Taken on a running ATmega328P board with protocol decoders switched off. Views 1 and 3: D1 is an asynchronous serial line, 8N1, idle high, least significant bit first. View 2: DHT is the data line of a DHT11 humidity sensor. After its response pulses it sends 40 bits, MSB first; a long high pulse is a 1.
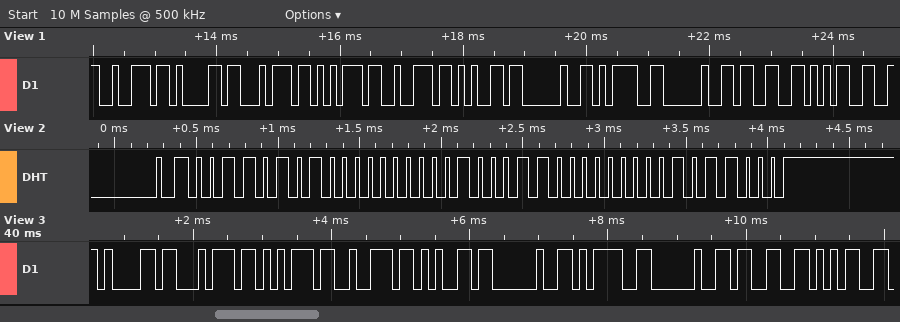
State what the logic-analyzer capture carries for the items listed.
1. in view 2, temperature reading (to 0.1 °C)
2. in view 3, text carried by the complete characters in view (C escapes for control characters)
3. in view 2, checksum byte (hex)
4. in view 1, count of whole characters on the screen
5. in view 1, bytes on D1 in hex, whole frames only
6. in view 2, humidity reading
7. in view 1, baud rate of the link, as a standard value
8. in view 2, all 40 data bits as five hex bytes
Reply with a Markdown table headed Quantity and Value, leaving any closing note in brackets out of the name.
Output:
| Quantity | Value |
|---|---|
| in view 2, temperature reading | 35.0 °C |
| in view 3, text carried by the complete characters in view | "ature = 35" |
| in view 2, checksum byte | 0x58 |
| in view 1, count of whole characters on the screen | 11 |
| in view 1, bytes on D1 in hex, whole frames only | 72 61 74 75 72 65 20 3D 20 33 35 |
| in view 2, humidity reading | 53 % |
| in view 1, baud rate of the link, as a standard value | 9600 baud |
| in view 2, all 40 data bits as five hex bytes | 35 00 23 00 58 |
